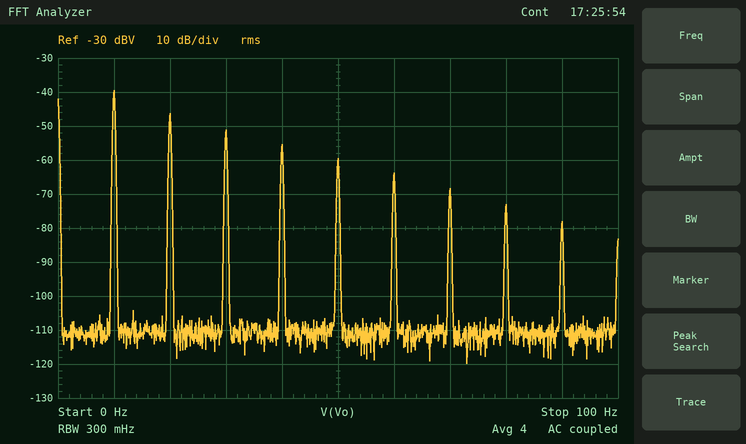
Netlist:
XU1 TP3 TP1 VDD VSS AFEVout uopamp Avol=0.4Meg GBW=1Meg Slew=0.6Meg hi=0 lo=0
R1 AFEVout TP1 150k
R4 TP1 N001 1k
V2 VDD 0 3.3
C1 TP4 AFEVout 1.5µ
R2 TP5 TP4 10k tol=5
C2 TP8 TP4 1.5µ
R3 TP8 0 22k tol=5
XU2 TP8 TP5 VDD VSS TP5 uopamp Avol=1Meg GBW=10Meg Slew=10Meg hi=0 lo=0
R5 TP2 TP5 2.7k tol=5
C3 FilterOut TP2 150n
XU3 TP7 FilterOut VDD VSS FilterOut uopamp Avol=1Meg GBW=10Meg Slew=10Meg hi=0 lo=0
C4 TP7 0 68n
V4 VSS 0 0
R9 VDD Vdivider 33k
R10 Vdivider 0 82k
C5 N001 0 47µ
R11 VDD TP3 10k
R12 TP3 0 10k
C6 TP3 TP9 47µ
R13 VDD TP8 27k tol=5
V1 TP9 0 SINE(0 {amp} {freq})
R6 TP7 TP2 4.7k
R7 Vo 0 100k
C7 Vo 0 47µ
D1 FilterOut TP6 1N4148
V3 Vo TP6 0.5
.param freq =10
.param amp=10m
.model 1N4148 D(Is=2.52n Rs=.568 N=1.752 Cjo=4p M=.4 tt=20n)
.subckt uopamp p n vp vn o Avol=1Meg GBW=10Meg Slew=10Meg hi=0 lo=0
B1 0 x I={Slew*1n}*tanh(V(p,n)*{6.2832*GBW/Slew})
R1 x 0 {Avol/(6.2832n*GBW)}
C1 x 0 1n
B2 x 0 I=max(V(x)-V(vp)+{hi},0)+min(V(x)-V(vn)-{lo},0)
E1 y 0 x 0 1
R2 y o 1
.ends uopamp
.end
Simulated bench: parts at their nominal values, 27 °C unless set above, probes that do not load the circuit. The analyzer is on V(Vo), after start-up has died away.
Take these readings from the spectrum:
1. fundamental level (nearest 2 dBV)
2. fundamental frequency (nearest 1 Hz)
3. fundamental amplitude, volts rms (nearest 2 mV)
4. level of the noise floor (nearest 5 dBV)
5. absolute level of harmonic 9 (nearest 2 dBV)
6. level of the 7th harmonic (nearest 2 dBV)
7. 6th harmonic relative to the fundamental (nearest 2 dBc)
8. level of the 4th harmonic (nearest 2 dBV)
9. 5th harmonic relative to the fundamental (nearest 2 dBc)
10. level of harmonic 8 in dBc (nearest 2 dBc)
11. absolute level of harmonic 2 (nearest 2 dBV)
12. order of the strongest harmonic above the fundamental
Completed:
-40 dBV
10 Hz
10 mV
-110 dBV
-78 dBV
-68 dBV
-24 dBc
-56 dBV
-20 dBc
-34 dBc
-46 dBV
2
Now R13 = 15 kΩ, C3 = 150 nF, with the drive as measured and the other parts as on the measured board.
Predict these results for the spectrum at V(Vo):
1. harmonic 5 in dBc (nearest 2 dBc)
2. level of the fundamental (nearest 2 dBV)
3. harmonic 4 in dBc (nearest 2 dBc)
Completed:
-22 dBc
-38 dBV
-18 dBc
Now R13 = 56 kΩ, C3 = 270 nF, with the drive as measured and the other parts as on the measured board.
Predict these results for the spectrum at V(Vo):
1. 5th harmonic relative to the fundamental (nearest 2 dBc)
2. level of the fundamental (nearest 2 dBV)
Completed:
-18 dBc
-40 dBV
